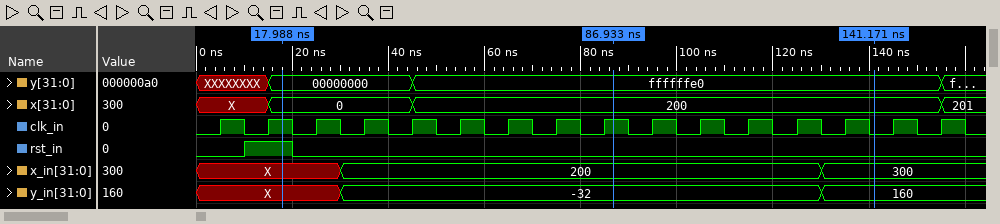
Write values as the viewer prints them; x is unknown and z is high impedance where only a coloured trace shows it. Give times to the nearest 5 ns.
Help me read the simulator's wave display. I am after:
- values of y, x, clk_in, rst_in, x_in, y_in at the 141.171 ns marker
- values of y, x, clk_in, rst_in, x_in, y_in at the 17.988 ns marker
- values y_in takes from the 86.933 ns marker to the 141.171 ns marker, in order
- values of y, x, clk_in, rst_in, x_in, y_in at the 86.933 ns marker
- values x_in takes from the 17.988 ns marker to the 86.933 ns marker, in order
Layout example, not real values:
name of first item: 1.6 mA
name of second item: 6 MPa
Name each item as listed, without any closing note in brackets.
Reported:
values of y, x, clk_in, rst_in, x_in, y_in at the 141.171 ns marker: y=ffffffe0, x=200, clk_in=0, rst_in=0, x_in=300, y_in=160
values of y, x, clk_in, rst_in, x_in, y_in at the 17.988 ns marker: y=00000000, x=0, clk_in=1, rst_in=1, x_in=X, y_in=X
values y_in takes from the 86.933 ns marker to the 141.171 ns marker, in order: -32, 160
values of y, x, clk_in, rst_in, x_in, y_in at the 86.933 ns marker: y=ffffffe0, x=200, clk_in=1, rst_in=0, x_in=200, y_in=-32
values x_in takes from the 17.988 ns marker to the 86.933 ns marker, in order: X, 200
